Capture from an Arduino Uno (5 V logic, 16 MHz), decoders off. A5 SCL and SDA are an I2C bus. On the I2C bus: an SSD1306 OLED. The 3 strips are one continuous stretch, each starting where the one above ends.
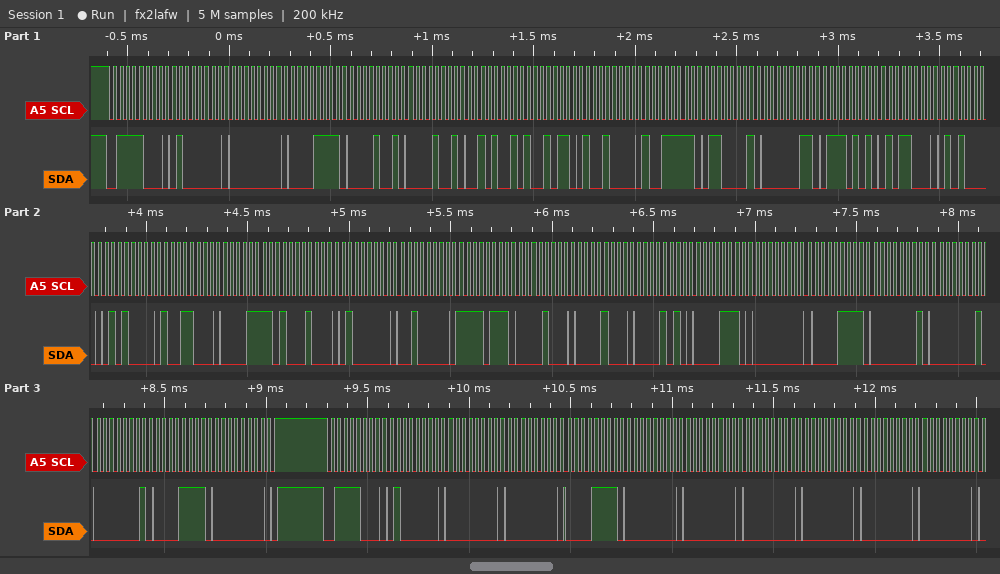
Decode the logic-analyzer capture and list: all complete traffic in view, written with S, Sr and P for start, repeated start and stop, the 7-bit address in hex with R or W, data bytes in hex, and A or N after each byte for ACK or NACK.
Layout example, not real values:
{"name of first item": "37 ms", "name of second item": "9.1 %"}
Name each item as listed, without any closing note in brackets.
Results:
{"all complete traffic in view, written with S, Sr and P for start, repeated start and stop, the 7-bit address in hex with R or W, data bytes in hex, and A or N after each byte for ACK or NACK": "S 3CW A 40 A 00 A 0F A 09 A 09 A 29 A 96 A 90 A 9F A 61 A 03 A 75 A 58 A 50 A 50 A 98 A 0F A 88 A 40 A 20 A F7 A 08 A 08 A 0A A 0E A 00 A 0F A 01 A 01 A 01 A 0F A 00 A P S 3CW A 40 A 00 A 00 A 0F A 00 A 00 A 00 A 00 A 00 A 00 A"}
